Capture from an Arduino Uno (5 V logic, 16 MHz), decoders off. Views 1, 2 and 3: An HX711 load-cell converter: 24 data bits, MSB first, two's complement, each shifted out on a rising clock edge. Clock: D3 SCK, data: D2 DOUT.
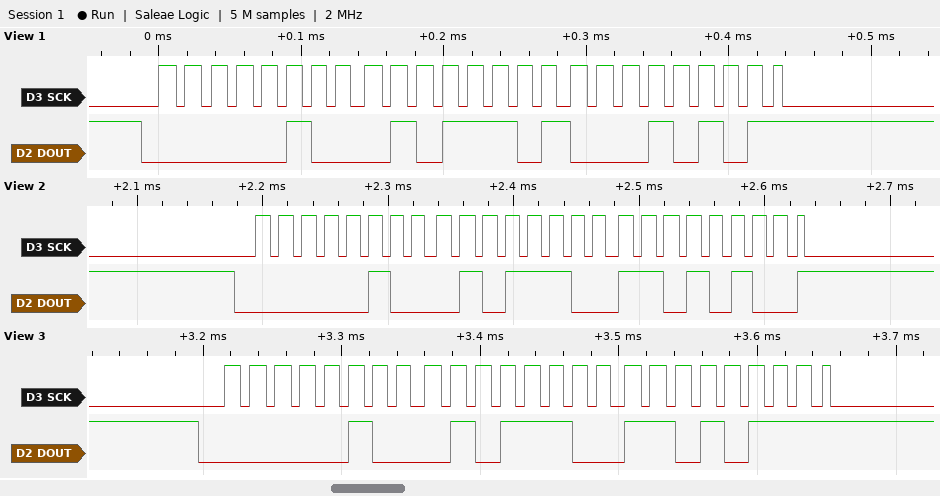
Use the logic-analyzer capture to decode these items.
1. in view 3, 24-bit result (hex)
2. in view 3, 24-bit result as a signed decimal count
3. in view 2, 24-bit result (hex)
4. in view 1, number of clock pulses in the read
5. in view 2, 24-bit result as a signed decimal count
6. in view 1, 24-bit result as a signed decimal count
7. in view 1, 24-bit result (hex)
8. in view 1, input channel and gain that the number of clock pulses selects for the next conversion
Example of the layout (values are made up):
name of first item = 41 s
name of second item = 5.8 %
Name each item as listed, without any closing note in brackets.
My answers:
in view 3, 24-bit result = 0x045CD7
in view 3, 24-bit result as a signed decimal count = 285911
in view 2, 24-bit result = 0x045CD4
in view 1, number of clock pulses in the read = 25
in view 2, 24-bit result as a signed decimal count = 285908
in view 1, 24-bit result as a signed decimal count = 285973
in view 1, 24-bit result = 0x045D15
in view 1, input channel and gain that the number of clock pulses selects for the next conversion = channel A, gain 128
